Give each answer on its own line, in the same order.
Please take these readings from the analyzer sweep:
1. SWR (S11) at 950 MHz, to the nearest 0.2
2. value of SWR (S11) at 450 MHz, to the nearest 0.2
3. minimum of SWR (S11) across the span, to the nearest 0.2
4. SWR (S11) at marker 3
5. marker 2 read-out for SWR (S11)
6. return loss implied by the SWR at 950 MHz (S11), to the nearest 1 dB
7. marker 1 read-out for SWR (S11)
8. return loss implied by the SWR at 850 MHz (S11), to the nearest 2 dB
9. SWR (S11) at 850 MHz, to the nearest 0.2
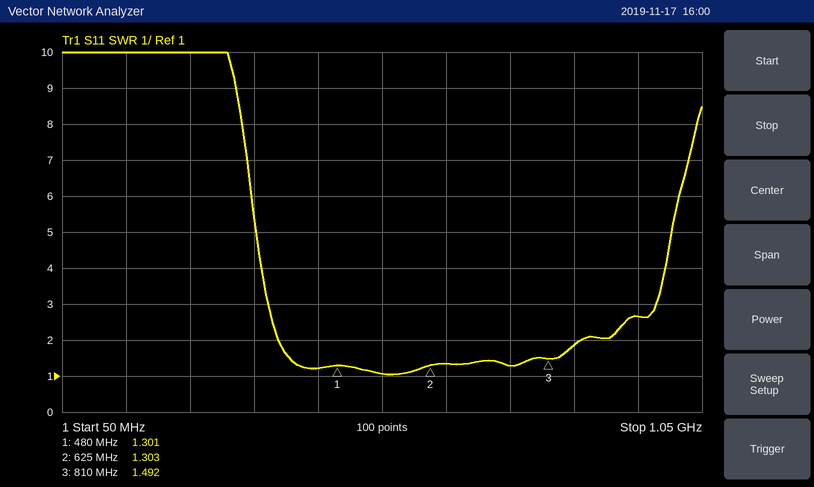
2.6
1.2
1.0
1.492
1.303
7 dB
1.301
10 dB
1.8
